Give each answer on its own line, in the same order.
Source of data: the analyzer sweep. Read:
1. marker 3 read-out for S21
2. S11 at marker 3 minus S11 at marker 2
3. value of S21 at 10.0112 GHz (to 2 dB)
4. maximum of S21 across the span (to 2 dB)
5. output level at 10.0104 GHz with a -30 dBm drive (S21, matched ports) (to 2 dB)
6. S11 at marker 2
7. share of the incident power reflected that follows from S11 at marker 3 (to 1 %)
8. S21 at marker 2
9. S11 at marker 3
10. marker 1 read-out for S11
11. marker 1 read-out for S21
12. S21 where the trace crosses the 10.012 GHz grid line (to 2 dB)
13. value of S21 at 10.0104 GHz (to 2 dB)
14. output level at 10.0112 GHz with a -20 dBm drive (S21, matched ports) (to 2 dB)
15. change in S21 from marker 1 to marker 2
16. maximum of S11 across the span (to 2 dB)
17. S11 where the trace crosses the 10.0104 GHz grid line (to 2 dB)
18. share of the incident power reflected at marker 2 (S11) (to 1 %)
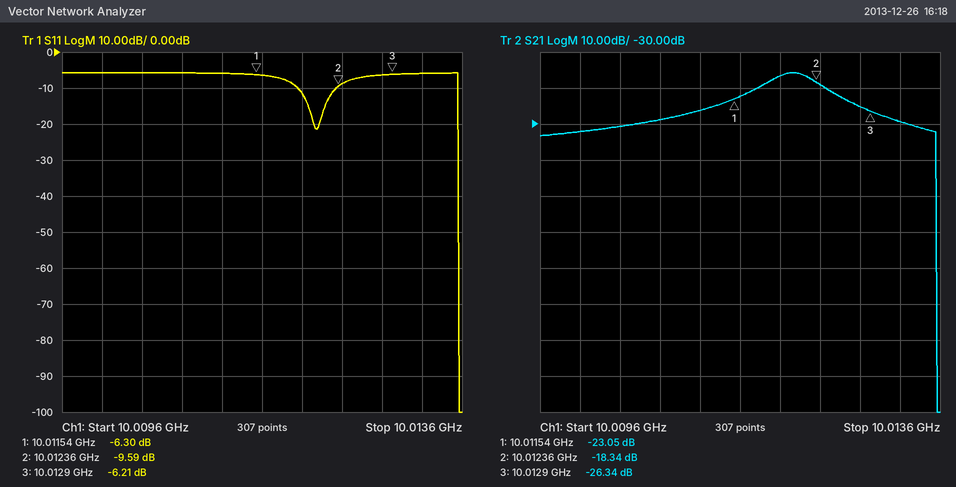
-26.34 dB
3.38 dB
-26 dB
-16 dB
-60 dBm
-9.59 dB
24 %
-18.34 dB
-6.21 dB
-6.30 dB
-23.05 dB
-16 dB
-30 dB
-46 dBm
4.71 dB
-6 dB
-6 dB
11 %
